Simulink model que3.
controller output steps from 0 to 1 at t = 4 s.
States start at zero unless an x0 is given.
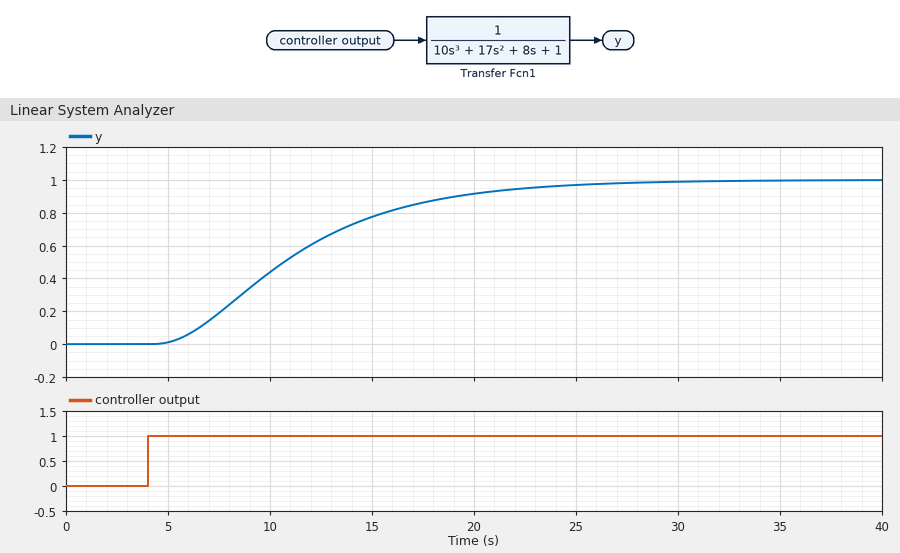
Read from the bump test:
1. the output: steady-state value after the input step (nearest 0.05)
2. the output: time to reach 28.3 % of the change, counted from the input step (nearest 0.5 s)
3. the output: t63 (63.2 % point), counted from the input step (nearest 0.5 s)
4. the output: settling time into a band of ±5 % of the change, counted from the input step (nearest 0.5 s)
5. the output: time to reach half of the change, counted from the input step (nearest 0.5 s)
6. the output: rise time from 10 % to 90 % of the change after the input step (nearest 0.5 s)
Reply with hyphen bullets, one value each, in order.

- 1.00
- 4.5 s
- 8.5 s
- 18.5 s
- 6.5 s
- 12.5 s
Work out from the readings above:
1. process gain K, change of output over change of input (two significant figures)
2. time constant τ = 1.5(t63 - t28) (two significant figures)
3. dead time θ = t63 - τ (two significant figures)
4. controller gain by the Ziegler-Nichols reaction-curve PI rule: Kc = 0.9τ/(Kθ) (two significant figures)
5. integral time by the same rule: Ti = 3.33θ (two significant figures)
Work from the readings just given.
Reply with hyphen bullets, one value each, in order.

- 1.0
- 6.0 s
- 2.5 s
- 2.2
- 8.3 s
